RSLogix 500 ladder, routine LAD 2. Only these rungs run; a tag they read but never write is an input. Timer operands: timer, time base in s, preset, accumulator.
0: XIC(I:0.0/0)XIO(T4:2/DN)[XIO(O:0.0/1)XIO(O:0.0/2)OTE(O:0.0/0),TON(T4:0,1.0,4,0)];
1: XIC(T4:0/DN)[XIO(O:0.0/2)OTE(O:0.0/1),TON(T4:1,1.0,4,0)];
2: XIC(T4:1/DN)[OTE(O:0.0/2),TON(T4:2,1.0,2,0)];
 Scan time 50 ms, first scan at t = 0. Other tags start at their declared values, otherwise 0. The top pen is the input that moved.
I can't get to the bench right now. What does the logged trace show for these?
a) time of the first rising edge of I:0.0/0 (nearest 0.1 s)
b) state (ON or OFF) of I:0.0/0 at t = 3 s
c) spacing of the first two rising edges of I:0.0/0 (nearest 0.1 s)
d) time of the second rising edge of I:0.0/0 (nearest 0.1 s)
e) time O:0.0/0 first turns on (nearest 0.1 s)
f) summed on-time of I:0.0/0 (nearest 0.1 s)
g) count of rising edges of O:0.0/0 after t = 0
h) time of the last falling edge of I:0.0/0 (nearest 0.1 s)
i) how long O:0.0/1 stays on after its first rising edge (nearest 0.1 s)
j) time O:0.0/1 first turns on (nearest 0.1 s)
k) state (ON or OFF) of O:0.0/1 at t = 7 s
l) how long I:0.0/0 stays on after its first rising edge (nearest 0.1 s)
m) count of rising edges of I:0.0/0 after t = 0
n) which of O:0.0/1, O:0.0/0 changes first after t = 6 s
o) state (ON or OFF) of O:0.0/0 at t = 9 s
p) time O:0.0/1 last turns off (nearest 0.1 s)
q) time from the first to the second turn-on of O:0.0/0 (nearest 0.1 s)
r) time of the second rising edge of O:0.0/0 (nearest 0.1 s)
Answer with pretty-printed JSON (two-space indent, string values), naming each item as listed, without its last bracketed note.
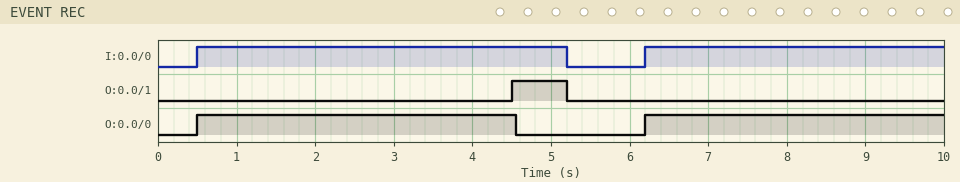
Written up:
{
  "time of the first rising edge of I:0.0/0": "0.5 s",
  "state (ON or OFF) of I:0.0/0 at t = 3 s": "ON",
  "spacing of the first two rising edges of I:0.0/0": "5.7 s",
  "time of the second rising edge of I:0.0/0": "6.2 s",
  "time O:0.0/0 first turns on": "0.5 s",
  "summed on-time of I:0.0/0": "8.5 s",
  "count of rising edges of O:0.0/0 after t = 0": "2",
  "time of the last falling edge of I:0.0/0": "5.2 s",
  "how long O:0.0/1 stays on after its first rising edge": "0.7 s",
  "time O:0.0/1 first turns on": "4.5 s",
  "state (ON or OFF) of O:0.0/1 at t = 7 s": "OFF",
  "how long I:0.0/0 stays on after its first rising edge": "4.7 s",
  "count of rising edges of I:0.0/0 after t = 0": "2",
  "which of O:0.0/1, O:0.0/0 changes first after t = 6 s": "O:0.0/0",
  "state (ON or OFF) of O:0.0/0 at t = 9 s": "ON",
  "time O:0.0/1 last turns off": "5.2 s",
  "time from the first to the second turn-on of O:0.0/0": "5.7 s",
  "time of the second rising edge of O:0.0/0": "6.2 s"
}
